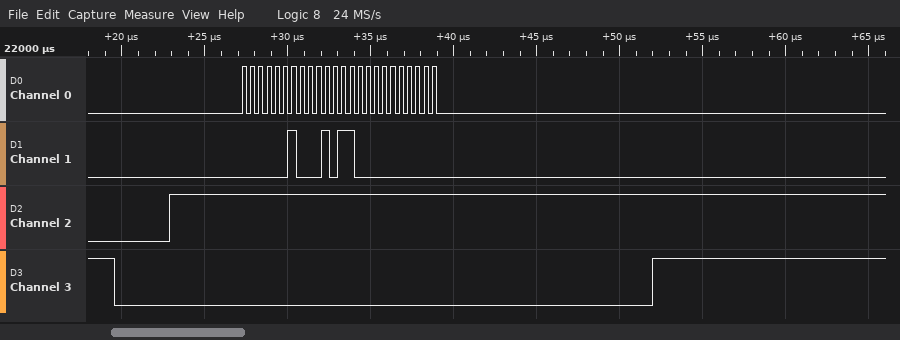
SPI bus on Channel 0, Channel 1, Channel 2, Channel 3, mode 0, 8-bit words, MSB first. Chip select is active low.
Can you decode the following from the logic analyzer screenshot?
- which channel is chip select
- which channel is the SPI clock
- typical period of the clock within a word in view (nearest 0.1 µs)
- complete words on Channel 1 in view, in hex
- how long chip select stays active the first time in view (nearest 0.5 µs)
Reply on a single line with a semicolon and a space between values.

Channel 3; Channel 0; 0.5 µs; 02, 2C, 00; 32.5 µs
